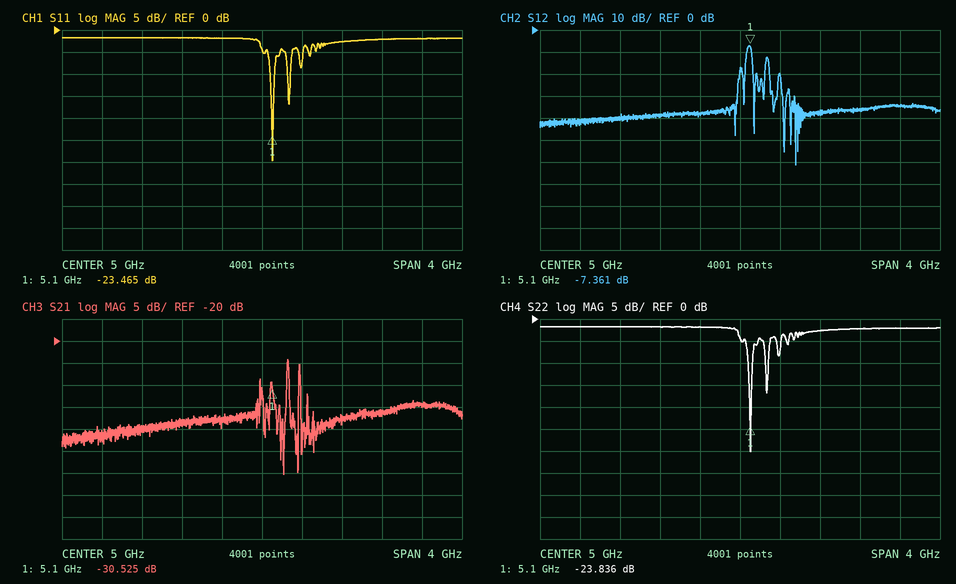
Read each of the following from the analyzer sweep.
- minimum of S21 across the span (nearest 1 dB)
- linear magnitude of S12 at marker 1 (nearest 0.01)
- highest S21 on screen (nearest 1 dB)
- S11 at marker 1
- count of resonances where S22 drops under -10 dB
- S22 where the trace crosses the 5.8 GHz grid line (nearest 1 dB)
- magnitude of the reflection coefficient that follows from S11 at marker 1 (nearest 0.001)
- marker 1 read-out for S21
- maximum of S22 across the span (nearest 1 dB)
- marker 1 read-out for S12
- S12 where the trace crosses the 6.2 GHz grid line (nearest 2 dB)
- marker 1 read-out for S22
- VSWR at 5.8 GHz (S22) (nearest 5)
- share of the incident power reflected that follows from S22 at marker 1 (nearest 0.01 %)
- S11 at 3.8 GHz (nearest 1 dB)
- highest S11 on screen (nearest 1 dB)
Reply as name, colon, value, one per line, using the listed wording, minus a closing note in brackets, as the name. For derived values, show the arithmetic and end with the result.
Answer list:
minimum of S21 across the span: -50 dB
linear magnitude of S12 at marker 1: 10^(-7.361/20) ≈ 0.43
highest S21 on screen: -24 dB
S11 at marker 1: -23.465 dB
count of resonances where S22 drops under -10 dB: 2
S22 where the trace crosses the 5.8 GHz grid line: -3 dB
magnitude of the reflection coefficient that follows from S11 at marker 1: 10^(-23.465/20) ≈ 0.067
marker 1 read-out for S21: -30.525 dB
maximum of S22 across the span: -2 dB
marker 1 read-out for S12: -7.361 dB
S12 where the trace crosses the 6.2 GHz grid line: -36 dB
marker 1 read-out for S22: -23.836 dB
VSWR at 5.8 GHz (S22): |Γ| = 10^(-3/20) = 0.7079; VSWR = (1 + 0.7079)/(1 − 0.7079) ≈ 5.85, so 5 to the nearest 5
share of the incident power reflected that follows from S22 at marker 1: 10^(-23.836/10) ≈ 0.41 %
S11 at 3.8 GHz: -2 dB
highest S11 on screen: -2 dB
